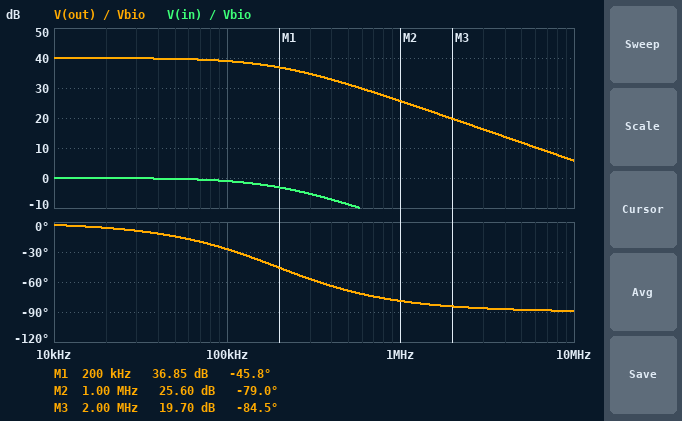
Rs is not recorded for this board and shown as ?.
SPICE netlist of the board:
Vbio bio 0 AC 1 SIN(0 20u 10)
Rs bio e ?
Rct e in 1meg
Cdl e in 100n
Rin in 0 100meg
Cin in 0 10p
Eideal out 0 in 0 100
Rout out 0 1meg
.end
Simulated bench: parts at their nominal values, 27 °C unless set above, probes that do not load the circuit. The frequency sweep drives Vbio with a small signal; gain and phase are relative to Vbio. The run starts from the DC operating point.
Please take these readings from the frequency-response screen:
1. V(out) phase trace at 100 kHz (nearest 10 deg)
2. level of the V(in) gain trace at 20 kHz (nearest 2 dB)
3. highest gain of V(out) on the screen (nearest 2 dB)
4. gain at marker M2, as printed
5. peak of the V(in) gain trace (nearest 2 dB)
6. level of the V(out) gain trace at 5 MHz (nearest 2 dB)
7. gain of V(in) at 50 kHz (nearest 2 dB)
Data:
-30 deg
0 dB
40 dB
25.60 dB
0 dB
12 dB
0 dB
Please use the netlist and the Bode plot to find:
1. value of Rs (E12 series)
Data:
82 kΩ
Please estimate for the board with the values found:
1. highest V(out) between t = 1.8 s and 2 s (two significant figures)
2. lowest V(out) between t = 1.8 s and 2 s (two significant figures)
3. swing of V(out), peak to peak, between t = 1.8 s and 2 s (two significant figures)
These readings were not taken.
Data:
2.0 mV
-2.0 mV
4.0 mV
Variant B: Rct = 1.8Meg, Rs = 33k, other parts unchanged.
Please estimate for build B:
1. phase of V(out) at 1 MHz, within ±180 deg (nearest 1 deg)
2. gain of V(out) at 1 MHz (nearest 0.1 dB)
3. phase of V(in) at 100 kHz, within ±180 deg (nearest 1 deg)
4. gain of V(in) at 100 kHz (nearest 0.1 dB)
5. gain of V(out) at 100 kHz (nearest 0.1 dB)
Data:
-64 deg
32.8 dB
-12 deg
-0.2 dB
39.8 dB
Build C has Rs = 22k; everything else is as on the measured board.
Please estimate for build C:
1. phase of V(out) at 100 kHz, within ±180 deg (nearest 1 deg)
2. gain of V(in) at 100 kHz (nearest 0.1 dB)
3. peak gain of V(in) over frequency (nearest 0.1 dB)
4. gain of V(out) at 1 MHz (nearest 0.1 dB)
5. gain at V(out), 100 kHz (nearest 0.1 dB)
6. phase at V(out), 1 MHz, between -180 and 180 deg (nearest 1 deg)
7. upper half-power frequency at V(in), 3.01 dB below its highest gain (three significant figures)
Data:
-8 deg
-0.1 dB
0 dB
35.4 dB
39.9 dB
-54 deg
724 kHz
